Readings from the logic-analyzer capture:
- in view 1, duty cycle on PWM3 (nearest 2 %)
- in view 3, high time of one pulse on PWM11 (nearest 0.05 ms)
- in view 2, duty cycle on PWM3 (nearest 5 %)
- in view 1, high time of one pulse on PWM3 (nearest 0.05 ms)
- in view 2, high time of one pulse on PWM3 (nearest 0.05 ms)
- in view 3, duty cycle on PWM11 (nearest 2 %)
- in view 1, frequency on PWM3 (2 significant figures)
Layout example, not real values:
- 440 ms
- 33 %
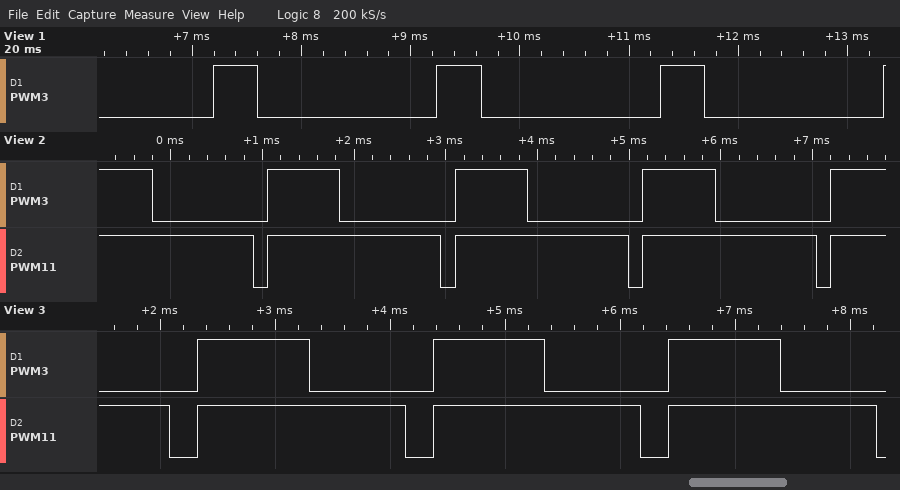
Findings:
- 20 %
- 1.80 ms
- 40 %
- 0.40 ms
- 0.80 ms
- 88 %
- 490 Hz
